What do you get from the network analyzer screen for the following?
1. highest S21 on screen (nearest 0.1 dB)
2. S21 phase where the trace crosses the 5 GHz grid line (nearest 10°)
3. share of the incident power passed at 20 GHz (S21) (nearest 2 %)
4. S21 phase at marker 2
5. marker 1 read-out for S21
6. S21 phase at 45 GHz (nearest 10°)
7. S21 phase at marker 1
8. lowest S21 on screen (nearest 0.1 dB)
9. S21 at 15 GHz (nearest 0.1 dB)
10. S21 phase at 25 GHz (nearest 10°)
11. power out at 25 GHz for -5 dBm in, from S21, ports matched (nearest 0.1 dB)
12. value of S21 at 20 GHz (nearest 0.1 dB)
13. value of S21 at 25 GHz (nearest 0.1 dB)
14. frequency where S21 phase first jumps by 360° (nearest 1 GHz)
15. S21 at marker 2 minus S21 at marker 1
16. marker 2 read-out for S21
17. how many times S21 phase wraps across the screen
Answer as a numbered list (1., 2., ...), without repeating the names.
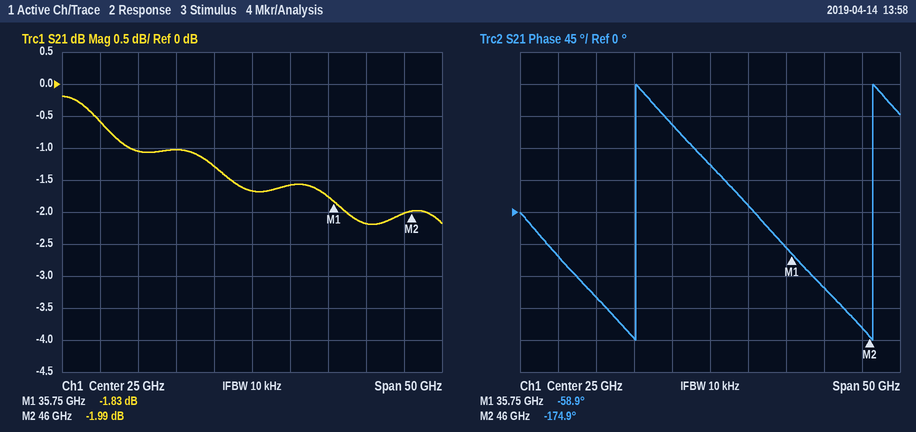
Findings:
1. -0.2 dB
2. -60°
3. 74 %
4. -174.9°
5. -1.83 dB
6. -160°
7. -58.9°
8. -2.2 dB
9. -1.0 dB
10. 70°
11. -6.7 dBm
12. -1.3 dB
13. -1.7 dB
14. 15 GHz
15. -0.16 dB
16. -1.99 dB
17. 2
